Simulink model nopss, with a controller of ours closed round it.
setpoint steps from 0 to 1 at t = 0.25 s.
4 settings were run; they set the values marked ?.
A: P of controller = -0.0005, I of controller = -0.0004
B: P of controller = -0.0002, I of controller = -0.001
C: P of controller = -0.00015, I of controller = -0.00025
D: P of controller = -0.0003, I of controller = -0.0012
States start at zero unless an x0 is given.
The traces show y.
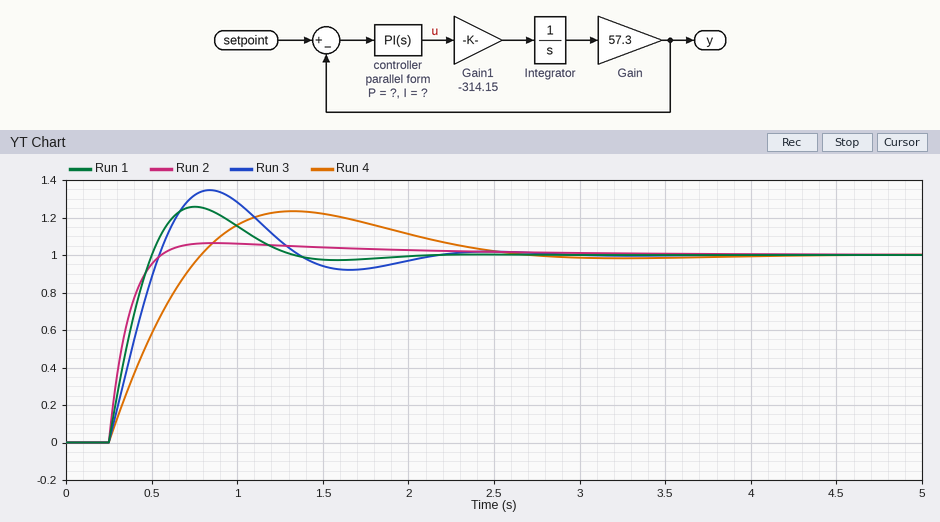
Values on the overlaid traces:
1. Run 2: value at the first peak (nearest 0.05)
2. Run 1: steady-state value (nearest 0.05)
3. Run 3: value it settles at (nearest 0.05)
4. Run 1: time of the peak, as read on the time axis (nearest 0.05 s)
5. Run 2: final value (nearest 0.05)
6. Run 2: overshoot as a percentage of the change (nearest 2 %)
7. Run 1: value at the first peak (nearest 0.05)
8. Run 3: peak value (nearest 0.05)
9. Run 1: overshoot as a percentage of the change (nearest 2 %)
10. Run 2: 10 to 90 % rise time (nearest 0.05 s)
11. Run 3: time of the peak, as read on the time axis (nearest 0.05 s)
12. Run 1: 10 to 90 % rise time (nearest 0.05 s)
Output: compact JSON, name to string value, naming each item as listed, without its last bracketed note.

{"Run 2: value at the first peak": "1.05", "Run 1: steady-state value": "1.00", "Run 3: value it settles at": "1.00", "Run 1: time of the peak, as read on the time axis": "0.75 s", "Run 2: final value": "1.00", "Run 2: overshoot as a percentage of the change": "6 %", "Run 1: value at the first peak": "1.25", "Run 3: peak value": "1.35", "Run 1: overshoot as a percentage of the change": "26 %", "Run 2: 10 to 90 % rise time": "0.20 s", "Run 3: time of the peak, as read on the time axis": "0.85 s", "Run 1: 10 to 90 % rise time": "0.20 s"}
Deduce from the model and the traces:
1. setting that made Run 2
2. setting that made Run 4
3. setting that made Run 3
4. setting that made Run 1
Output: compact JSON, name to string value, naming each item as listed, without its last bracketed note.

{"setting that made Run 2": "A", "setting that made Run 4": "C", "setting that made Run 3": "B", "setting that made Run 1": "D"}
